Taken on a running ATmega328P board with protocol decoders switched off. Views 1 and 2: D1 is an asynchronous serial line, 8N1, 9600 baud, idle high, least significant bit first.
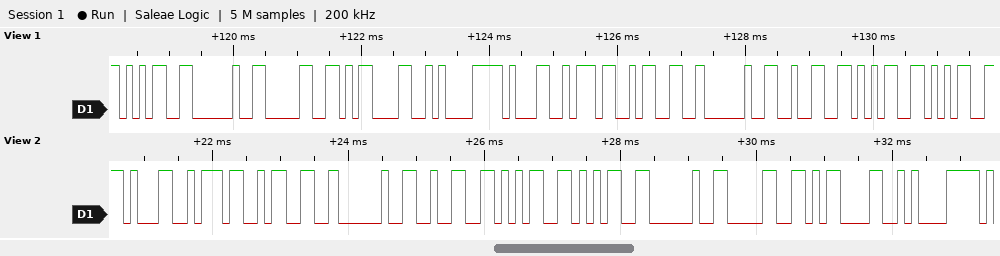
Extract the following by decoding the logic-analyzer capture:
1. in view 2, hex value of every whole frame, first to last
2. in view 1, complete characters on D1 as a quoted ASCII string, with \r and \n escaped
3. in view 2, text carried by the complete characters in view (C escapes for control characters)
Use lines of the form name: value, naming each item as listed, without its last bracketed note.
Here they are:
in view 2, hex value of every whole frame, first to last: 0x31 0x37 0x33 0x20 0x32 0x35 0x35 0x20 0x30 0x0D 0x0A
in view 1, complete characters on D1 as a quoted ASCII string, with \r and \n escaped: "5 0\r\n173 255"
in view 2, text carried by the complete characters in view: "173 255 0\r\n"
